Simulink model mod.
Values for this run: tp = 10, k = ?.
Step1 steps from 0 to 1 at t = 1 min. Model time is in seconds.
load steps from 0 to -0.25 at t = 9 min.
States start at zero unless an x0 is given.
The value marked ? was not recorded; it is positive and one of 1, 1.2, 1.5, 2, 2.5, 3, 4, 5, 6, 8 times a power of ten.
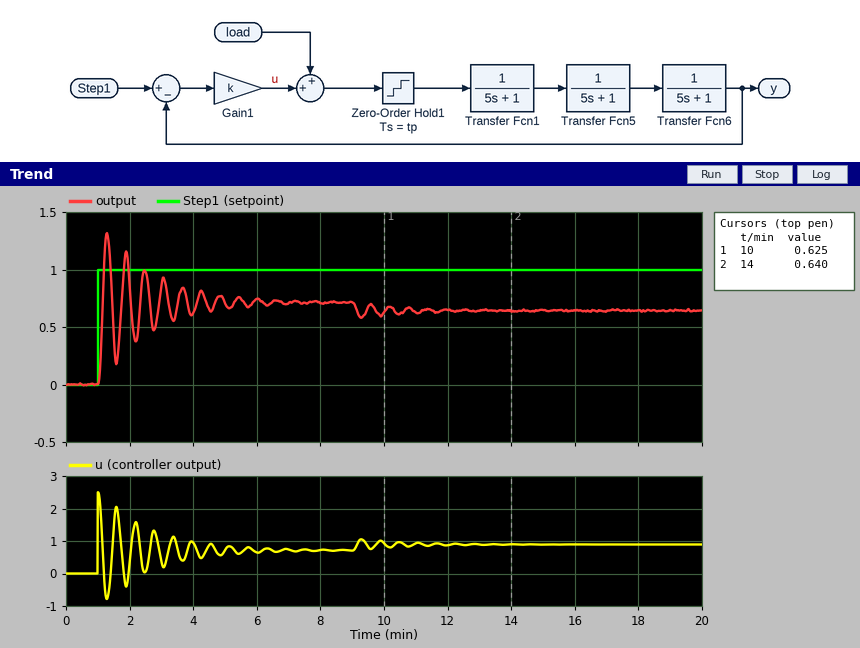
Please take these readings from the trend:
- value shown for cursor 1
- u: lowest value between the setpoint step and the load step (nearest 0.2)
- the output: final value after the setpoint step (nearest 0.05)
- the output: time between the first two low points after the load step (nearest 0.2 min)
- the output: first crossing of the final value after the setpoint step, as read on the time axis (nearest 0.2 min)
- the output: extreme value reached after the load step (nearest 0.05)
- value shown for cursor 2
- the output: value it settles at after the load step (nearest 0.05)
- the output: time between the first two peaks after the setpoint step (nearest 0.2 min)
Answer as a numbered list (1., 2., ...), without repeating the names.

1. 0.625
2. -0.8
3. 0.70
4. 0.6 min
5. 1.2 min
6. 0.60
7. 0.640
8. 0.65
9. 0.6 min
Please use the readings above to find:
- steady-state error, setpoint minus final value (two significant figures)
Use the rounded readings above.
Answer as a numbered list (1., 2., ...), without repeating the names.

1. 0.30
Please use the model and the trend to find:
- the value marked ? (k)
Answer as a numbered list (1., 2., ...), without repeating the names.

1. 2.5
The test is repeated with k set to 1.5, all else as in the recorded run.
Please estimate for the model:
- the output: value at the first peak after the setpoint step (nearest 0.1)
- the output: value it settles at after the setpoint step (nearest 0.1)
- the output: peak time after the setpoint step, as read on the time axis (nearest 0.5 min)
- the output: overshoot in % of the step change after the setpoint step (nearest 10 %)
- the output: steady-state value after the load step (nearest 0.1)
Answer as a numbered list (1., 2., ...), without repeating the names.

1. 0.9
2. 0.6
3. 1.5 min
4. 50 %
5. 0.5
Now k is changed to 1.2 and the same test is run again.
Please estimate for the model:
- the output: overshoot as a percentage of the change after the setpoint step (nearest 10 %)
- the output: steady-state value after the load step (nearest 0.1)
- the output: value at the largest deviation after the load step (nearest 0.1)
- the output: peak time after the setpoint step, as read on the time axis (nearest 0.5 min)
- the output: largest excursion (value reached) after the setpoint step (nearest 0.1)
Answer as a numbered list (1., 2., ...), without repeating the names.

1. 40 %
2. 0.4
3. 0.4
4. 1.5 min
5. 0.8
